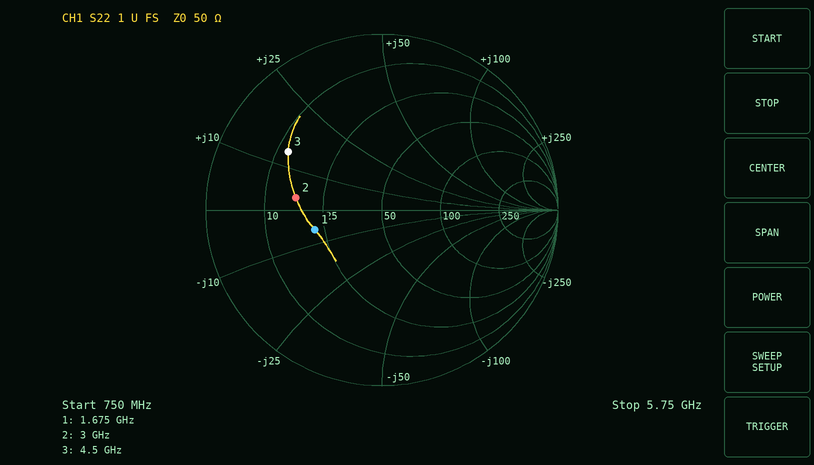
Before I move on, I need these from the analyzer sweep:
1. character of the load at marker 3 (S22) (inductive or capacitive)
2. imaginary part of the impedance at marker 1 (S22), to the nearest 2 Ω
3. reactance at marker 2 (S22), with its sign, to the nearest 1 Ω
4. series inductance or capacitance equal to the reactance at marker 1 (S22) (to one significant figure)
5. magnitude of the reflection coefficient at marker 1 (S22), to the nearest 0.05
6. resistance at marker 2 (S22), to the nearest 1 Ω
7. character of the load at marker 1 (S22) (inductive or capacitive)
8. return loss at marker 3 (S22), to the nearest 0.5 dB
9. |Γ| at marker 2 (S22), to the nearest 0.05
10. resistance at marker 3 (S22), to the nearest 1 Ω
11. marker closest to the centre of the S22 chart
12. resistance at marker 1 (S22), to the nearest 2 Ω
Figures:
inductive
-6 Ω
+3 Ω
20 pF
0.40
17 Ω
capacitive
4.0 dB
0.50
12 Ω
marker 1
22 Ω
